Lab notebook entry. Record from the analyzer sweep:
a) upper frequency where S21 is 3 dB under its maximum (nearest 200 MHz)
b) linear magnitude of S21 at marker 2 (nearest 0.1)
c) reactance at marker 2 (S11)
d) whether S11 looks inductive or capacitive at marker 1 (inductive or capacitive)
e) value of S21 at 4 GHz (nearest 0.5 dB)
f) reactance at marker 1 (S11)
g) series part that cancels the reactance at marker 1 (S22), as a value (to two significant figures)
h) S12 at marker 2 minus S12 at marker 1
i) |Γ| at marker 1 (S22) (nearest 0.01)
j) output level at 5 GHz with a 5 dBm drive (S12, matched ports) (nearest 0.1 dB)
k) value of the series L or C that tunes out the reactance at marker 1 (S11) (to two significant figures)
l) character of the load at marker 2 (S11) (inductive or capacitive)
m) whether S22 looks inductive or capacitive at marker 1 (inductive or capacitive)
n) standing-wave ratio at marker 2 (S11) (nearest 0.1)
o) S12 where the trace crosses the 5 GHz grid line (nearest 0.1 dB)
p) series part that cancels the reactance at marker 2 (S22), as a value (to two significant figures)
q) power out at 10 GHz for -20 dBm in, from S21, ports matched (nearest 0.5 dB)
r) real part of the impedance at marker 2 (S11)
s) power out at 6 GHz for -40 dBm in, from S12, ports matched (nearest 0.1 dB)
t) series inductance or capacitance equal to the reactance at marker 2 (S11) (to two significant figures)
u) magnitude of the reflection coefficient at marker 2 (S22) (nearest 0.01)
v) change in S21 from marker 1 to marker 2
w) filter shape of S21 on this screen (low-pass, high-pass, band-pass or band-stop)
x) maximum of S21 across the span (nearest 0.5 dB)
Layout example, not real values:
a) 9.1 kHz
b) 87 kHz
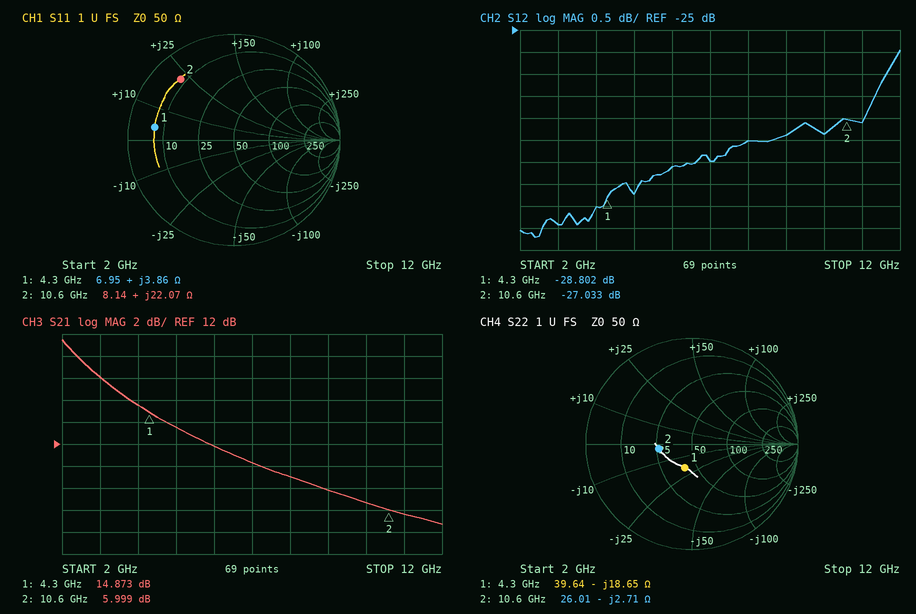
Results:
a) 2.8 GHz
b) 2.0
c) +22.07 Ω
d) inductive
e) 15.5 dB
f) +3.86 Ω
g) 690 pH
h) 1.769 dB
i) 0.23
j) -23.7 dBm
k) 9.6 pF
l) inductive
m) capacitive
n) 7.4
o) -28.7 dB
p) 41 pH
q) -13.5 dBm
r) 8.14 Ω
s) -68.1 dBm
t) 330 pH
u) 0.32
v) -8.874 dB
w) low-pass
x) 21.5 dB
